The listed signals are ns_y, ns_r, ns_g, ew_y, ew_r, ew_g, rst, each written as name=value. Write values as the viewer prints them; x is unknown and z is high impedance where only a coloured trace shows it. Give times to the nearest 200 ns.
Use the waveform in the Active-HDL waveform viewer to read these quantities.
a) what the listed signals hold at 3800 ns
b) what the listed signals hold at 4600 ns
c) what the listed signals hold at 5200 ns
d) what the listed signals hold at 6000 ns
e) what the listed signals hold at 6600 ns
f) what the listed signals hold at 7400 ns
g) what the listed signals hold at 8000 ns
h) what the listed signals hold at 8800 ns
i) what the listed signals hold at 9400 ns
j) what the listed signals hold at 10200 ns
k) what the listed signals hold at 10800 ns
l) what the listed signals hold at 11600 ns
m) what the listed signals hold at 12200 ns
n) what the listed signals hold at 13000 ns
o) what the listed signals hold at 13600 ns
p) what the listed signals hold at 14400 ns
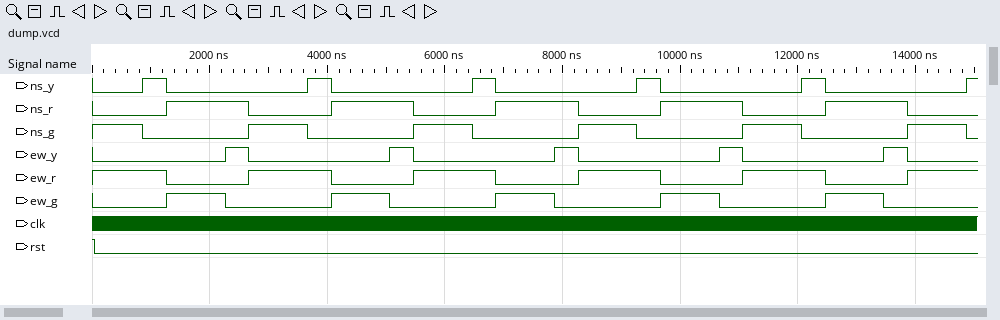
ns_y=1, ns_r=0, ns_g=0, ew_y=0, ew_r=1, ew_g=0, rst=0
ns_y=0, ns_r=1, ns_g=0, ew_y=0, ew_r=0, ew_g=1, rst=0
ns_y=0, ns_r=1, ns_g=0, ew_y=1, ew_r=0, ew_g=0, rst=0
ns_y=0, ns_r=0, ns_g=1, ew_y=0, ew_r=1, ew_g=0, rst=0
ns_y=1, ns_r=0, ns_g=0, ew_y=0, ew_r=1, ew_g=0, rst=0
ns_y=0, ns_r=1, ns_g=0, ew_y=0, ew_r=0, ew_g=1, rst=0
ns_y=0, ns_r=1, ns_g=0, ew_y=1, ew_r=0, ew_g=0, rst=0
ns_y=0, ns_r=0, ns_g=1, ew_y=0, ew_r=1, ew_g=0, rst=0
ns_y=1, ns_r=0, ns_g=0, ew_y=0, ew_r=1, ew_g=0, rst=0
ns_y=0, ns_r=1, ns_g=0, ew_y=0, ew_r=0, ew_g=1, rst=0
ns_y=0, ns_r=1, ns_g=0, ew_y=1, ew_r=0, ew_g=0, rst=0
ns_y=0, ns_r=0, ns_g=1, ew_y=0, ew_r=1, ew_g=0, rst=0
ns_y=1, ns_r=0, ns_g=0, ew_y=0, ew_r=1, ew_g=0, rst=0
ns_y=0, ns_r=1, ns_g=0, ew_y=0, ew_r=0, ew_g=1, rst=0
ns_y=0, ns_r=1, ns_g=0, ew_y=1, ew_r=0, ew_g=0, rst=0
ns_y=0, ns_r=0, ns_g=1, ew_y=0, ew_r=1, ew_g=0, rst=0
